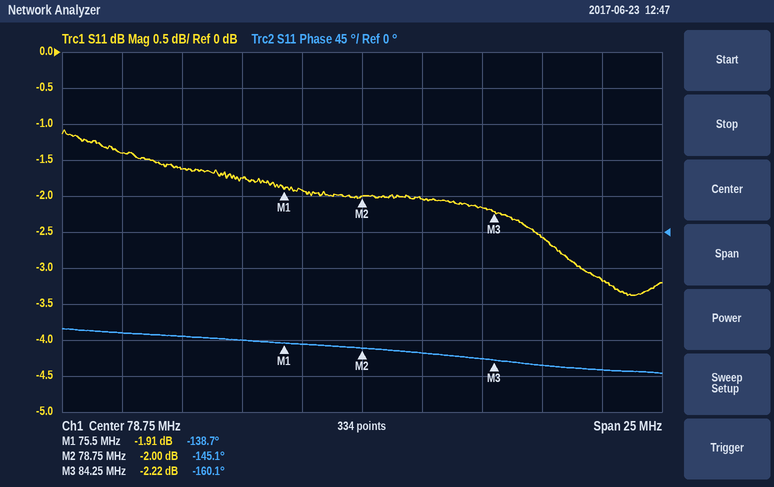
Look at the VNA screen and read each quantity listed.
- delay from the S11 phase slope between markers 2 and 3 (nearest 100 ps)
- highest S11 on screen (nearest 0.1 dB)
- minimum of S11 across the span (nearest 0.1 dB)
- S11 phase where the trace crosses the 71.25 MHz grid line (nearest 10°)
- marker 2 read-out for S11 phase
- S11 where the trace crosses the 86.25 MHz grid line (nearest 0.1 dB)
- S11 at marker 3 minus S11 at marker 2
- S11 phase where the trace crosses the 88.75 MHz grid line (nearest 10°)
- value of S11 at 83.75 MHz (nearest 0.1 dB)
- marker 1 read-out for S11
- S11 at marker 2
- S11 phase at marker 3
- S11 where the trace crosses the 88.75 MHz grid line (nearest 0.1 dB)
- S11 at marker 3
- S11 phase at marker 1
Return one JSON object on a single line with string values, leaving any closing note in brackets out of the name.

{"delay from the S11 phase slope between markers 2 and 3": "7.6 ns", "highest S11 on screen": "-1.1 dB", "minimum of S11 across the span": "-3.4 dB", "S11 phase where the trace crosses the 71.25 MHz grid line": "-130°", "marker 2 read-out for S11 phase": "-145.1°", "S11 where the trace crosses the 86.25 MHz grid line": "-2.6 dB", "S11 at marker 3 minus S11 at marker 2": "-0.22 dB", "S11 phase where the trace crosses the 88.75 MHz grid line": "-170°", "value of S11 at 83.75 MHz": "-2.2 dB", "marker 1 read-out for S11": "-1.91 dB", "S11 at marker 2": "-2.00 dB", "S11 phase at marker 3": "-160.1°", "S11 where the trace crosses the 88.75 MHz grid line": "-3.2 dB", "S11 at marker 3": "-2.22 dB", "S11 phase at marker 1": "-138.7°"}
